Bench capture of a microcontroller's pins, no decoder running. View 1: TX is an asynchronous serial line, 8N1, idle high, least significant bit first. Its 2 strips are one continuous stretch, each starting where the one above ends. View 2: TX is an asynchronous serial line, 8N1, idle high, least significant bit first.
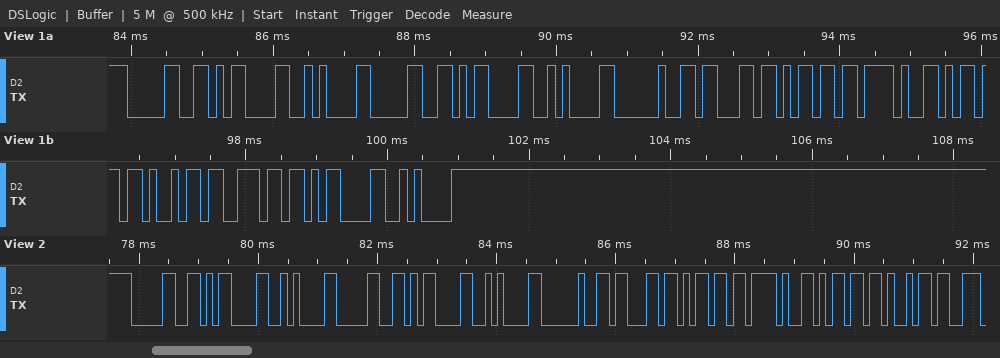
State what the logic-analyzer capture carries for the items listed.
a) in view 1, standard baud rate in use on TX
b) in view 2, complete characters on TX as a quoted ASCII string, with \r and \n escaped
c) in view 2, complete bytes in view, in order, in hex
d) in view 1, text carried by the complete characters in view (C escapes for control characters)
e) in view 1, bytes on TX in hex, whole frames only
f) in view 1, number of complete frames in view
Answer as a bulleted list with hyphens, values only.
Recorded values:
- 9600 baud
- "0\r\n0\r\n cm/mi"
- 30 0D 0A 30 0D 0A 20 63 6D 2F 6D 69
- "0\r\n0\r\n cm/min\r\n"
- 30 0D 0A 30 0D 0A 20 63 6D 2F 6D 69 6E 0D 0A
- 15
